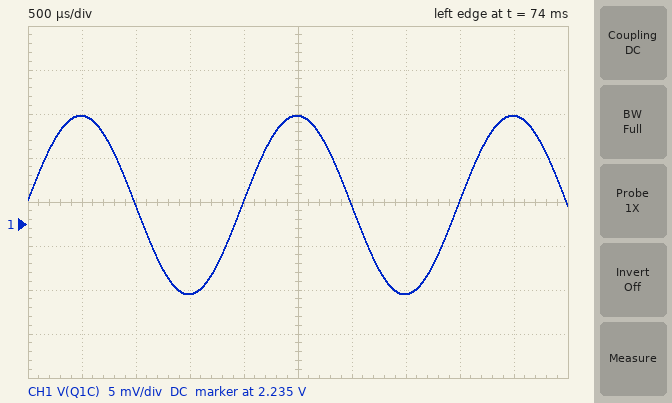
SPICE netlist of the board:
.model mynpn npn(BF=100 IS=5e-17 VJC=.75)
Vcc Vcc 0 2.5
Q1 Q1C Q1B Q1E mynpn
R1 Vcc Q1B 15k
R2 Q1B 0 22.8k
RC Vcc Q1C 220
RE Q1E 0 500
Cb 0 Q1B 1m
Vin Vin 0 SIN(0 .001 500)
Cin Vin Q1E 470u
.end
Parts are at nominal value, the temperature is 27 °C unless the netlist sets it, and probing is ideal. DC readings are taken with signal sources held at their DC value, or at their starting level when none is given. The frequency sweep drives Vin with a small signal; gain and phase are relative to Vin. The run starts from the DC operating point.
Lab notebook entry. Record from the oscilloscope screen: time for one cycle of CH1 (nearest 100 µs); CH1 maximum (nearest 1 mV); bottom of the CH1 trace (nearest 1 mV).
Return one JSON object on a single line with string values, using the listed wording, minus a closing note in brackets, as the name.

{"time for one cycle of CH1": "2.0 ms", "CH1 maximum": "2.247 V", "bottom of the CH1 trace": "2.227 V"}
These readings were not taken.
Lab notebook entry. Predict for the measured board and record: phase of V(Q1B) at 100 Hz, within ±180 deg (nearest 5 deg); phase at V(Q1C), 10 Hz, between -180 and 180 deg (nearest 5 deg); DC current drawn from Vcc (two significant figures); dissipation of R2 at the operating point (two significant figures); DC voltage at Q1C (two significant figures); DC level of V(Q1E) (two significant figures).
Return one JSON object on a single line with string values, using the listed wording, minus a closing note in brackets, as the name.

{"phase of V(Q1B) at 100 Hz, within ±180 deg": "-80 deg", "phase at V(Q1C), 10 Hz, between -180 and 180 deg": "60 deg", "DC current drawn from Vcc": "1.3 mA", "dissipation of R2 at the operating point": "86 µW", "DC voltage at Q1C": "2.2 V", "DC level of V(Q1E)": "600 mV"}
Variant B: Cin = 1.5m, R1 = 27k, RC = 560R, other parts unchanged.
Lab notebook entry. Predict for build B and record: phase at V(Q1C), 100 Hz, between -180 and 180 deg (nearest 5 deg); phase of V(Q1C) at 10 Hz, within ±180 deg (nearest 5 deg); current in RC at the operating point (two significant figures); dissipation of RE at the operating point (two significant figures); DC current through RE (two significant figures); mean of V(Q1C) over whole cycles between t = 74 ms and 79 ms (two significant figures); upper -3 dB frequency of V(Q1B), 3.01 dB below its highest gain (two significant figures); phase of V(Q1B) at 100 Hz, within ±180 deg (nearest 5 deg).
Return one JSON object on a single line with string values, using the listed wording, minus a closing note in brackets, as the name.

{"phase at V(Q1C), 100 Hz, between -180 and 180 deg": "0 deg", "phase of V(Q1C) at 10 Hz, within ±180 deg": "15 deg", "current in RC at the operating point": "580 µA", "dissipation of RE at the operating point": "170 µW", "DC current through RE": "590 µA", "mean of V(Q1C) over whole cycles between t = 74 ms and 79 ms": "2.2 V", "upper -3 dB frequency of V(Q1B), 3.01 dB below its highest gain": "2.7 Hz", "phase of V(Q1B) at 100 Hz, within ±180 deg": "-90 deg"}
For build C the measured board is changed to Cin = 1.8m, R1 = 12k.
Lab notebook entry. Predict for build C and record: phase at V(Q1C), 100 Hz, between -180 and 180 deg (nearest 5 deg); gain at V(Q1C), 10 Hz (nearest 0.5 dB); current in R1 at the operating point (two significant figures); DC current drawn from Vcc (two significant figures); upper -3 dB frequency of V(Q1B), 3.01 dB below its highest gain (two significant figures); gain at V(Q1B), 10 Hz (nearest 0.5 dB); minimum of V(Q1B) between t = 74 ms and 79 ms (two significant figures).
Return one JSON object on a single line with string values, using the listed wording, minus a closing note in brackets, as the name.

{"phase at V(Q1C), 100 Hz, between -180 and 180 deg": "5 deg", "gain at V(Q1C), 10 Hz": "20.5 dB", "current in R1 at the operating point": "81 µA", "DC current drawn from Vcc": "1.5 mA", "upper -3 dB frequency of V(Q1B), 3.01 dB below its highest gain": "5.3 Hz", "gain at V(Q1B), 10 Hz": "-42.0 dB", "minimum of V(Q1B) between t = 74 ms and 79 ms": "1.5 V"}
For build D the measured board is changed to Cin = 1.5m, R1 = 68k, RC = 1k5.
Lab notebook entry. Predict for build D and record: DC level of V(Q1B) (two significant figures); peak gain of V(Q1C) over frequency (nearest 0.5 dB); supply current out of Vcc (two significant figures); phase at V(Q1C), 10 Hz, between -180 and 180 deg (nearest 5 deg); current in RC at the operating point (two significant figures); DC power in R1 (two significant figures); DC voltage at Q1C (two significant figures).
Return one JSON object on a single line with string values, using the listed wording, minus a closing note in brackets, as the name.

{"DC level of V(Q1B)": "630 mV", "peak gain of V(Q1C) over frequency": "-20.5 dB", "supply current out of Vcc": "29 µA", "phase at V(Q1C), 10 Hz, between -180 and 180 deg": "0 deg", "current in RC at the operating point": "1.7 µA", "DC power in R1": "52 µW", "DC voltage at Q1C": "2.5 V"}
